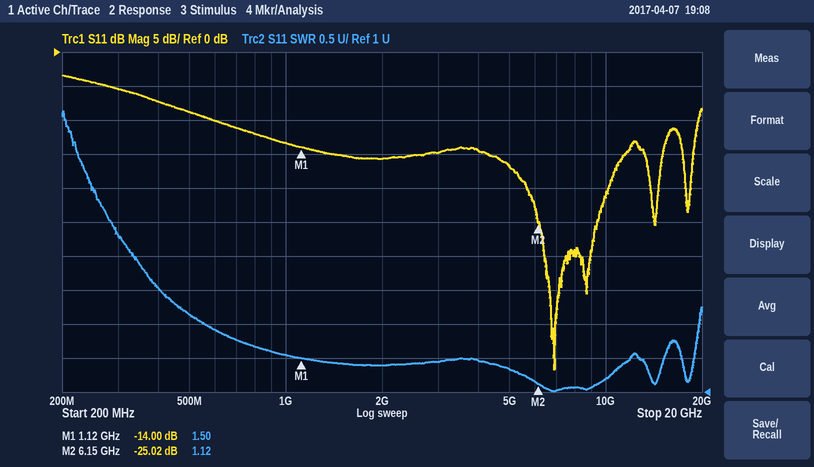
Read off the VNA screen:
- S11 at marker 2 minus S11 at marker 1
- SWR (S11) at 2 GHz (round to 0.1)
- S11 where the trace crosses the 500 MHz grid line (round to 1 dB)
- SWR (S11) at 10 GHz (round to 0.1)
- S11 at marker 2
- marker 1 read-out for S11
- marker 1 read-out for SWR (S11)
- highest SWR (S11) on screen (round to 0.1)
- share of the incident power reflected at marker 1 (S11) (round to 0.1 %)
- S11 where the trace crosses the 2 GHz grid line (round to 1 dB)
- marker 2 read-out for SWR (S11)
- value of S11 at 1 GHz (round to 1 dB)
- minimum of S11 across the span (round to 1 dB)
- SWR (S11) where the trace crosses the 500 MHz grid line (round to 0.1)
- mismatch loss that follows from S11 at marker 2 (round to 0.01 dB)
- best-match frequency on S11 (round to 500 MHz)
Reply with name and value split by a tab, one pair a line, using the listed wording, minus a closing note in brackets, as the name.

S11 at marker 2 minus S11 at marker 1	-11.02 dB
SWR (S11) at 2 GHz	1.4
S11 where the trace crosses the 500 MHz grid line	-9 dB
SWR (S11) at 10 GHz	1.2
S11 at marker 2	-25.02 dB
marker 1 read-out for S11	-14.00 dB
marker 1 read-out for SWR	1.50
highest SWR (S11) on screen	5.1
share of the incident power reflected at marker 1 (S11)	4.0 %
S11 where the trace crosses the 2 GHz grid line	-16 dB
marker 2 read-out for SWR	1.12
value of S11 at 1 GHz	-13 dB
minimum of S11 across the span	-47 dB
SWR (S11) where the trace crosses the 500 MHz grid line	2.1
mismatch loss that follows from S11 at marker 2	0.01 dB
best-match frequency on S11	7.0 GHz
